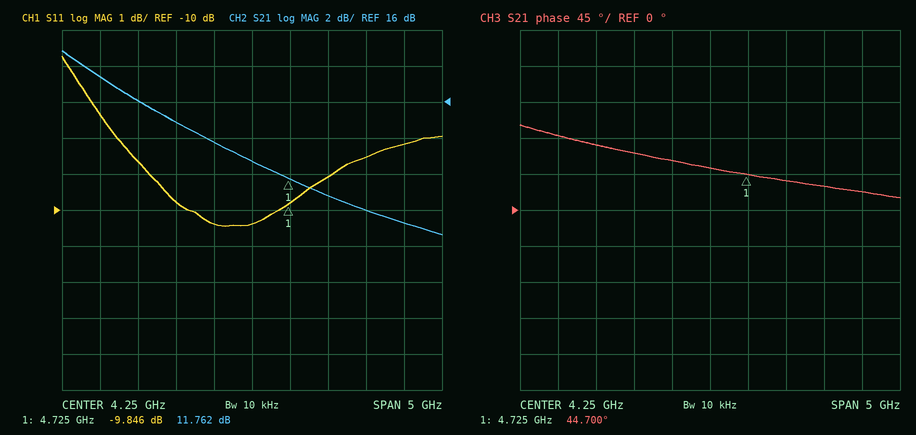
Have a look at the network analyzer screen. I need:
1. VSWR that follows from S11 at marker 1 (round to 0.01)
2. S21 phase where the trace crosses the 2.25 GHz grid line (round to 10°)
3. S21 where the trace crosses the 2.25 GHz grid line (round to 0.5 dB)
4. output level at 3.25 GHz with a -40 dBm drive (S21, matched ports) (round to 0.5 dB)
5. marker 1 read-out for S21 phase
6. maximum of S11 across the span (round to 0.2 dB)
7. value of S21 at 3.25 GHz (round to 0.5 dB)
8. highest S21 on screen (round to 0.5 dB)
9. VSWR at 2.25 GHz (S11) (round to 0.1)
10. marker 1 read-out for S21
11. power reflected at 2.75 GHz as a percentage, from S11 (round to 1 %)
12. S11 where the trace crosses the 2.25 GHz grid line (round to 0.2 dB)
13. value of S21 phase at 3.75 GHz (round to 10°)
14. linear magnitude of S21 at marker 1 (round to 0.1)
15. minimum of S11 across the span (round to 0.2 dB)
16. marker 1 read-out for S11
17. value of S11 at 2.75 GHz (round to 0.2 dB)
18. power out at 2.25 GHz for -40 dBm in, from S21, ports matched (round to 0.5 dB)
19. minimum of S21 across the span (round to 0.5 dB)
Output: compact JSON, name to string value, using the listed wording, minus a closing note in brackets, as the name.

{"VSWR that follows from S11 at marker 1": "1.95", "S21 phase where the trace crosses the 2.25 GHz grid line": "90°", "S21 where the trace crosses the 2.25 GHz grid line": "17.5 dB", "output level at 3.25 GHz with a -40 dBm drive (S21, matched ports)": "-25.0 dBm", "marker 1 read-out for S21 phase": "44.700°", "maximum of S11 across the span": "-5.8 dB", "value of S21 at 3.25 GHz": "15.0 dB", "highest S21 on screen": "19.0 dB", "VSWR at 2.25 GHz (S11)": "2.5", "marker 1 read-out for S21": "11.762 dB", "power reflected at 2.75 GHz as a percentage, from S11": "14 %", "S11 where the trace crosses the 2.25 GHz grid line": "-7.4 dB", "value of S21 phase at 3.75 GHz": "60°", "linear magnitude of S21 at marker 1": "3.9", "minimum of S11 across the span": "-10.4 dB", "marker 1 read-out for S11": "-9.846 dB", "value of S11 at 2.75 GHz": "-8.6 dB", "power out at 2.25 GHz for -40 dBm in, from S21, ports matched": "-22.5 dBm", "minimum of S21 across the span": "8.5 dB"}
